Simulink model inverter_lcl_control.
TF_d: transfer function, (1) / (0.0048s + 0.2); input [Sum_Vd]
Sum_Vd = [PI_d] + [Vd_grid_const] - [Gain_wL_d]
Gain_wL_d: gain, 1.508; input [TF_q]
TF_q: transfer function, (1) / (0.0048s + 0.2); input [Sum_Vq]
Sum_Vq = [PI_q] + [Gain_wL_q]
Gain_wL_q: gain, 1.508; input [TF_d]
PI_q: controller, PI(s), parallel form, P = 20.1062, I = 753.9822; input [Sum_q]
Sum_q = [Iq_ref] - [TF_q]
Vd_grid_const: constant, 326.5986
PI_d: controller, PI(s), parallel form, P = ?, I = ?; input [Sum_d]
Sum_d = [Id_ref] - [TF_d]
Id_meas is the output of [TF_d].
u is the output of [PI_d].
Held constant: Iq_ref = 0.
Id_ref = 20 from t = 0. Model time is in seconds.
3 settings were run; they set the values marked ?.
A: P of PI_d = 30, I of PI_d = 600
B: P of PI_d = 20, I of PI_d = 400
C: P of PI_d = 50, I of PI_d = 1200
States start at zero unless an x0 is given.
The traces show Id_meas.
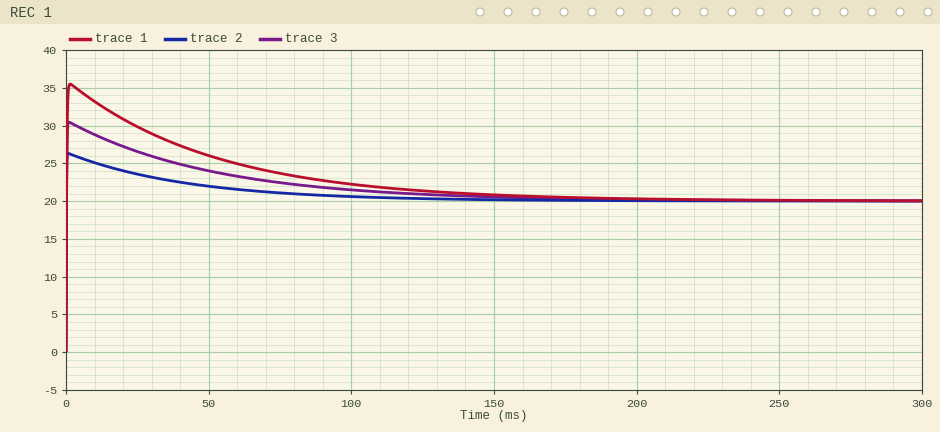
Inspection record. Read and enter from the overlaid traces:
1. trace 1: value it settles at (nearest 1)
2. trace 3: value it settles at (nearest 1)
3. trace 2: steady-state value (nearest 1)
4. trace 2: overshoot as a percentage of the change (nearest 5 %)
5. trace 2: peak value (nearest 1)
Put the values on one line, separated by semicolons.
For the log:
20; 20; 20; 30 %; 26
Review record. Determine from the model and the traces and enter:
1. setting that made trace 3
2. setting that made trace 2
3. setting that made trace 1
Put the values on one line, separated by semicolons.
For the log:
A; C; B
